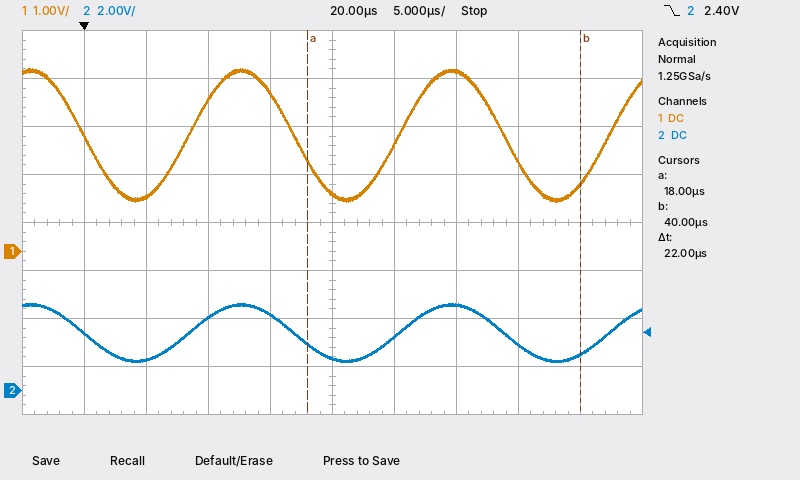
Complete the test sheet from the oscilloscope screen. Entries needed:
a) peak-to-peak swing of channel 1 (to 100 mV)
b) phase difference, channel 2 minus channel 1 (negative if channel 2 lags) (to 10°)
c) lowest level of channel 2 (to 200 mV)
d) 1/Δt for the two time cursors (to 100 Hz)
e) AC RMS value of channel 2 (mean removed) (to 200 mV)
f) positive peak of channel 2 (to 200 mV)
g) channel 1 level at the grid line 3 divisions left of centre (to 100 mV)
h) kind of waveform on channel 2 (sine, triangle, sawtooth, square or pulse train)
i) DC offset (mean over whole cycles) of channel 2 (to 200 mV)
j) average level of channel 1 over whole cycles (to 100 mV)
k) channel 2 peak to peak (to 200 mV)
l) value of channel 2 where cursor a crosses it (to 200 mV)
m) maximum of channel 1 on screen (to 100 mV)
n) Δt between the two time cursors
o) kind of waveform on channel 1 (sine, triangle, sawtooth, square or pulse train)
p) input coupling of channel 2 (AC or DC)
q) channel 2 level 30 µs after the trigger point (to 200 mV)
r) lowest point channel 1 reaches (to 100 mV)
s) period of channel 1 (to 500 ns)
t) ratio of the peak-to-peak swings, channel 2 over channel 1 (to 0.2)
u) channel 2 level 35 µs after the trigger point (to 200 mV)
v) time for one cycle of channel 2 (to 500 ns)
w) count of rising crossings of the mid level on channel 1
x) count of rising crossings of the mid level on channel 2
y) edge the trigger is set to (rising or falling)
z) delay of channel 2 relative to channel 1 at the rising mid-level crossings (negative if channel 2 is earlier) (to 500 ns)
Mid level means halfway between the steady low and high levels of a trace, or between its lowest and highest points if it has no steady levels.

2.8 V
0°
1.2 V
45.5 kHz
800 mV
3.6 V
1.1 V
sine
2.4 V
2.4 V
2.4 V
2.0 V
3.8 V
22 µs
sine
DC
3.6 V
1.0 V
17.0 µs
0.8
2.0 V
17.0 µs
3
3
falling
0.0 µs
